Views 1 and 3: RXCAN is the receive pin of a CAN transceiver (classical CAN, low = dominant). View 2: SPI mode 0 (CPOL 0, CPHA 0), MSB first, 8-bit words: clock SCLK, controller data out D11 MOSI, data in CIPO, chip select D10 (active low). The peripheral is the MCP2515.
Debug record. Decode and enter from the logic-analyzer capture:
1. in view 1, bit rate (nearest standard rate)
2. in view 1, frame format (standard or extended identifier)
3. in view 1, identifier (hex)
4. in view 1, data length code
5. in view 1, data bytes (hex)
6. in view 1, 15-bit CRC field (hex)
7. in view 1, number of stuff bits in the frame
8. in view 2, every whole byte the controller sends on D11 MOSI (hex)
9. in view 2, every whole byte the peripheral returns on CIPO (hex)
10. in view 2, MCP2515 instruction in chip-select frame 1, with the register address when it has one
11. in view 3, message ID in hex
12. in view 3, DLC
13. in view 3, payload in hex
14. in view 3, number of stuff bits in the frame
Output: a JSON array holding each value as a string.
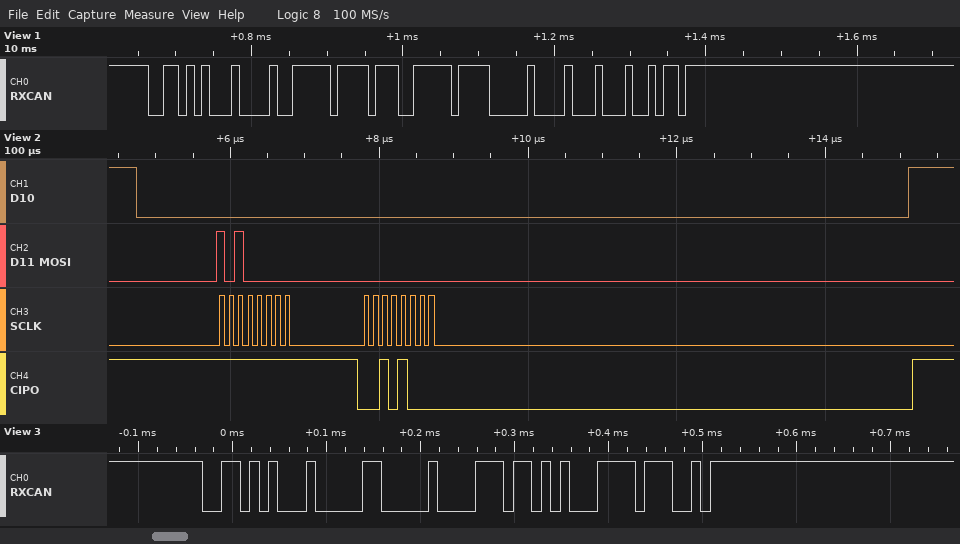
["100 kbit/s", "standard", "0x351", "4", "FF B9 FF 00", "0x2225", "3", "A0 00", "FF 28", "READ STATUS", "0x351", "2", "00 ED", "2"]
